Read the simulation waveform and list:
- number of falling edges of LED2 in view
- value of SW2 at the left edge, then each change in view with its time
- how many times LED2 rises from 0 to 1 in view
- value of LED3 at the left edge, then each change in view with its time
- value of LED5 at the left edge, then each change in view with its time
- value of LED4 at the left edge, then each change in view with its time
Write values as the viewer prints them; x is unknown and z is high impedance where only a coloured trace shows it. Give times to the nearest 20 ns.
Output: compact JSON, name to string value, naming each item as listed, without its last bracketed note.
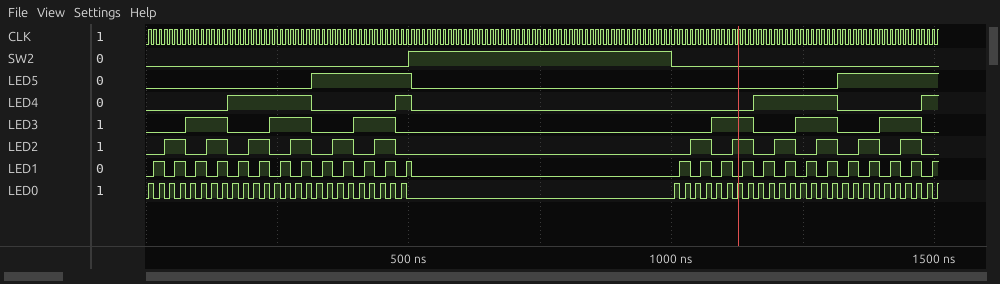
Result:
{"number of falling edges of LED2 in view": "12", "value of SW2 at the left edge, then each change in view with its time": "0, 1 at 500 ns, 0 at 1000 ns", "how many times LED2 rises from 0 to 1 in view": "12", "value of LED3 at the left edge, then each change in view with its time": "0, 1 at 80 ns, 0 at 160 ns, 1 at 240 ns, 0 at 320 ns, 1 at 400 ns, 0 at 480 ns, 1 at 1080 ns, 0 at 1160 ns, 1 at 1240 ns, 0 at 1320 ns, 1 at 1400 ns, 0 at 1480 ns", "value of LED5 at the left edge, then each change in view with its time": "0, 1 at 320 ns, 0 at 500 ns, 1 at 1320 ns", "value of LED4 at the left edge, then each change in view with its time": "0, 1 at 160 ns, 0 at 320 ns, 1 at 480 ns, 0 at 500 ns, 1 at 1160 ns, 0 at 1320 ns, 1 at 1480 ns"}
